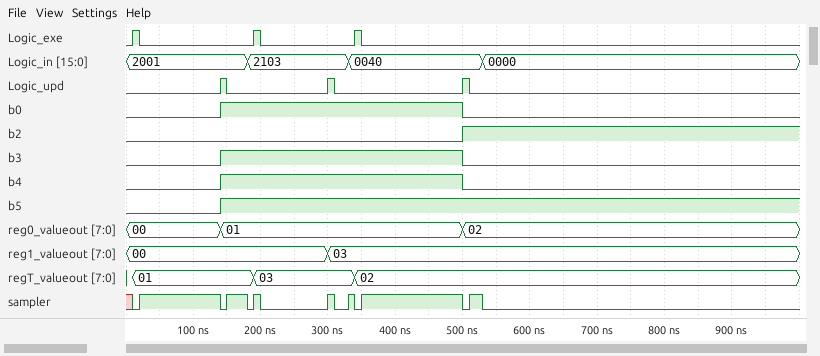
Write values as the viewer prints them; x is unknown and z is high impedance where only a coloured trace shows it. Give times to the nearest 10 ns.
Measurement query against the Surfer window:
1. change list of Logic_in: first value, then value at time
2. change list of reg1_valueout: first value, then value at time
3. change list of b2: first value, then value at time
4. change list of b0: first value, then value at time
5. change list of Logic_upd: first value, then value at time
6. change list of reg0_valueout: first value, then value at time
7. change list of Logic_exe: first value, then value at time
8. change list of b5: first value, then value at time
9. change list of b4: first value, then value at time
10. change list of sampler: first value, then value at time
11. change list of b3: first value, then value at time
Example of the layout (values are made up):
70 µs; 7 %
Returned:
2001, 2103 at 180 ns, 0040 at 330 ns, 0000 at 530 ns; 00, 03 at 300 ns; 0, 1 at 500 ns; 0, 1 at 140 ns, 0 at 500 ns; 0, 1 at 140 ns, 0 at 150 ns, 1 at 300 ns, 0 at 310 ns, 1 at 500 ns, 0 at 510 ns; 00, 01 at 140 ns, 02 at 500 ns; 0, 1 at 10 ns, 0 at 20 ns, 1 at 190 ns, 0 at 200 ns, 1 at 340 ns, 0 at 350 ns; 0, 1 at 140 ns; 0, 1 at 140 ns, 0 at 500 ns; x, 0 at 10 ns, 1 at 20 ns, 0 at 140 ns, 1 at 150 ns, 0 at 180 ns, 1 at 190 ns, 0 at 200 ns, 1 at 300 ns, 0 at 310 ns, 1 at 330 ns, 0 at 340 ns, 1 at 350 ns, 0 at 500 ns, 1 at 510 ns, 0 at 530 ns; 0, 1 at 140 ns, 0 at 500 ns
